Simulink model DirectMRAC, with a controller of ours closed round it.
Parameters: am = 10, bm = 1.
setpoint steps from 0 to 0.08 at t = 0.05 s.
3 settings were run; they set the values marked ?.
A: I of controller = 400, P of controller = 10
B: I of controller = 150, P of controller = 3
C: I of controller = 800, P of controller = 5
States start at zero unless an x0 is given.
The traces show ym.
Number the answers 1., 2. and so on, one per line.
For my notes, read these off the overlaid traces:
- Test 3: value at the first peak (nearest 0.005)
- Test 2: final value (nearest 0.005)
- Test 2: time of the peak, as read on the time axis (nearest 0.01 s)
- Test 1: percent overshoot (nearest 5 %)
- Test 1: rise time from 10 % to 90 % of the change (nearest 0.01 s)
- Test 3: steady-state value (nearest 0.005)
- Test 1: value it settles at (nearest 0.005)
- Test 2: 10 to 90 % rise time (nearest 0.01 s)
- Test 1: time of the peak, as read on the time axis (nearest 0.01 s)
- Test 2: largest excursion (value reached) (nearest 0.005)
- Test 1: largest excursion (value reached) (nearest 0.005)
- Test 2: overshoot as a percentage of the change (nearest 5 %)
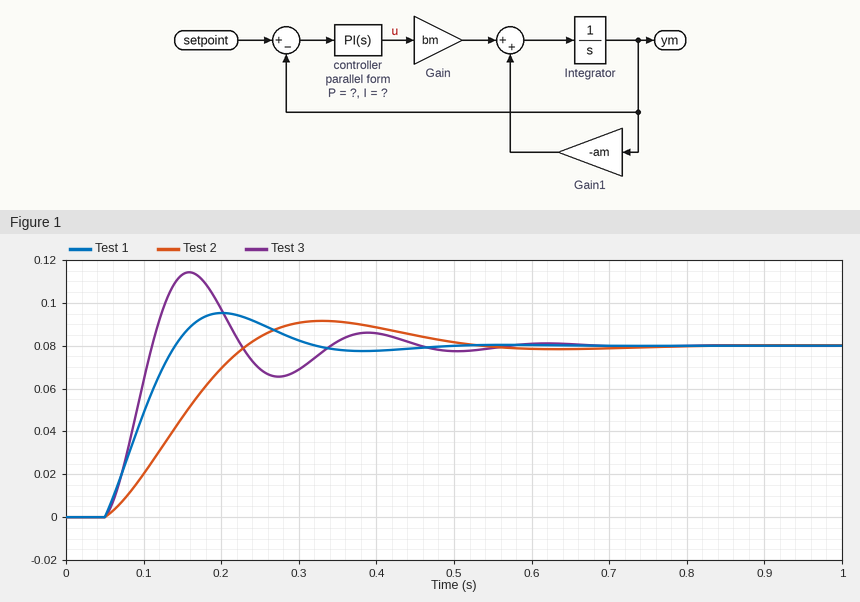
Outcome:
1. 0.115
2. 0.080
3. 0.33 s
4. 20 %
5. 0.07 s
6. 0.080
7. 0.080
8. 0.13 s
9. 0.20 s
10. 0.090
11. 0.095
12. 15 %
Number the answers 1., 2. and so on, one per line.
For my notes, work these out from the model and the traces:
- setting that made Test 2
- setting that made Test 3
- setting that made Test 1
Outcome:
1. B
2. C
3. A
